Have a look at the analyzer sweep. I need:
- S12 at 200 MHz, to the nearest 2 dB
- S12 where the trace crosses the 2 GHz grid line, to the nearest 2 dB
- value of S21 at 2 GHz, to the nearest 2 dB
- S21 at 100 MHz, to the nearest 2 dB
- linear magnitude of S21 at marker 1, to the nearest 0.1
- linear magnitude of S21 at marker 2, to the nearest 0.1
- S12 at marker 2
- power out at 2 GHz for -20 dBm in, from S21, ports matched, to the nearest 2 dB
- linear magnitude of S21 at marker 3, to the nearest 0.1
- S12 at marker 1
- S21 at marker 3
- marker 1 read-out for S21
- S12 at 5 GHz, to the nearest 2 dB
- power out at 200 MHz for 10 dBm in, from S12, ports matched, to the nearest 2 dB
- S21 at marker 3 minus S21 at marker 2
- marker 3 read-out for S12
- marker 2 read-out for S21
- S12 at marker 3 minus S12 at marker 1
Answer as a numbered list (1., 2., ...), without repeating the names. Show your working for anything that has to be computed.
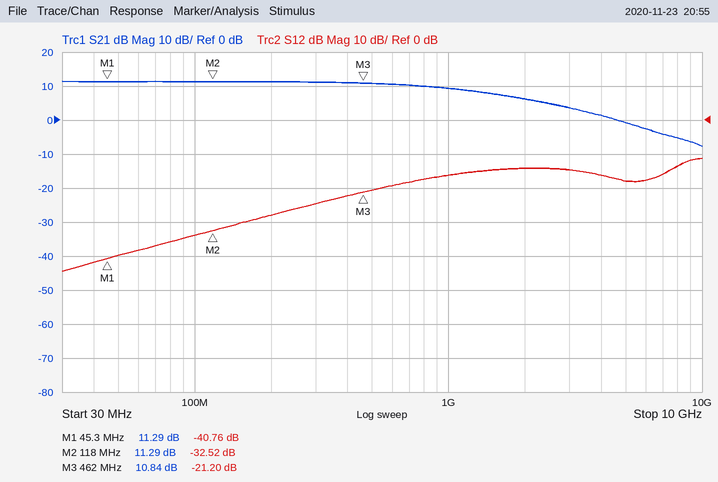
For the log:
1. -28 dB
2. -14 dB
3. 6 dB
4. 12 dB
5. 10^(11.29/20) ≈ 3.7
6. 10^(11.29/20) ≈ 3.7
7. -32.52 dB
8. -20 dBm + (6 dB) = -14 dBm
9. 10^(10.84/20) ≈ 3.5
10. -40.76 dB
11. 10.84 dB
12. 11.29 dB
13. -18 dB
14. 10 dBm + (-28 dB) = -18 dBm
15. 10.84 − (11.29) = -0.45 dB
16. -21.20 dB
17. 11.29 dB
18. -21.2 − (-40.76) = 19.56 dB
